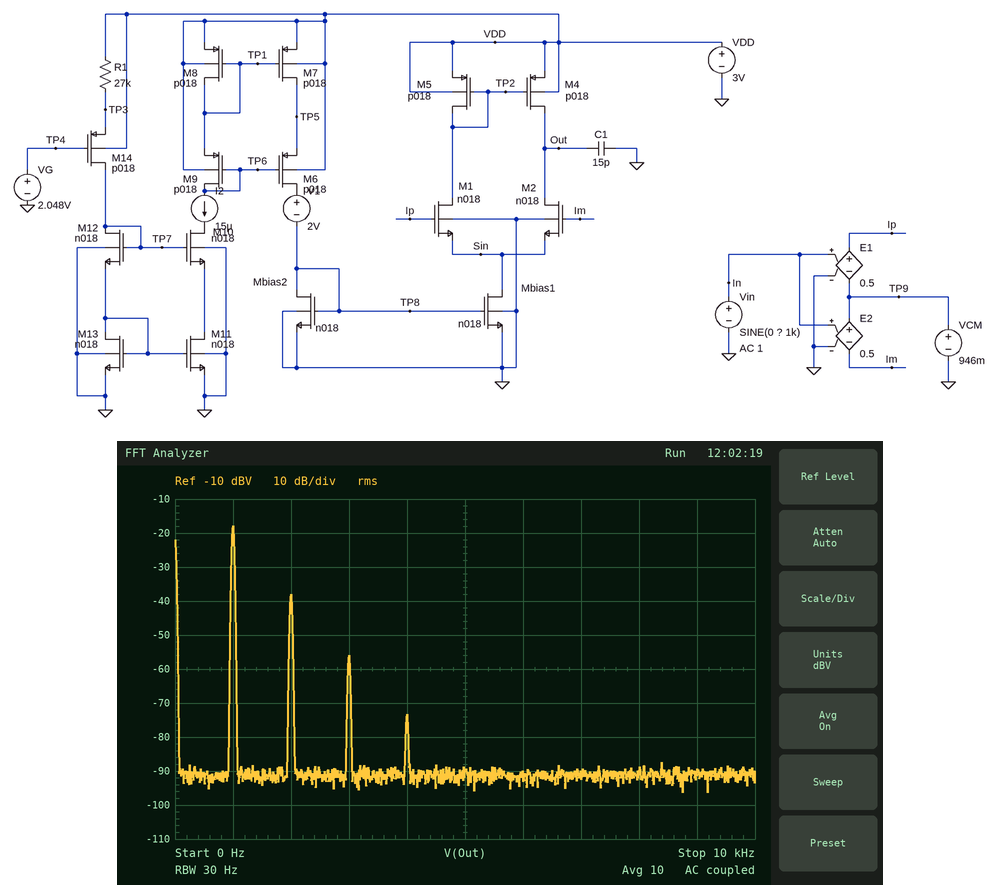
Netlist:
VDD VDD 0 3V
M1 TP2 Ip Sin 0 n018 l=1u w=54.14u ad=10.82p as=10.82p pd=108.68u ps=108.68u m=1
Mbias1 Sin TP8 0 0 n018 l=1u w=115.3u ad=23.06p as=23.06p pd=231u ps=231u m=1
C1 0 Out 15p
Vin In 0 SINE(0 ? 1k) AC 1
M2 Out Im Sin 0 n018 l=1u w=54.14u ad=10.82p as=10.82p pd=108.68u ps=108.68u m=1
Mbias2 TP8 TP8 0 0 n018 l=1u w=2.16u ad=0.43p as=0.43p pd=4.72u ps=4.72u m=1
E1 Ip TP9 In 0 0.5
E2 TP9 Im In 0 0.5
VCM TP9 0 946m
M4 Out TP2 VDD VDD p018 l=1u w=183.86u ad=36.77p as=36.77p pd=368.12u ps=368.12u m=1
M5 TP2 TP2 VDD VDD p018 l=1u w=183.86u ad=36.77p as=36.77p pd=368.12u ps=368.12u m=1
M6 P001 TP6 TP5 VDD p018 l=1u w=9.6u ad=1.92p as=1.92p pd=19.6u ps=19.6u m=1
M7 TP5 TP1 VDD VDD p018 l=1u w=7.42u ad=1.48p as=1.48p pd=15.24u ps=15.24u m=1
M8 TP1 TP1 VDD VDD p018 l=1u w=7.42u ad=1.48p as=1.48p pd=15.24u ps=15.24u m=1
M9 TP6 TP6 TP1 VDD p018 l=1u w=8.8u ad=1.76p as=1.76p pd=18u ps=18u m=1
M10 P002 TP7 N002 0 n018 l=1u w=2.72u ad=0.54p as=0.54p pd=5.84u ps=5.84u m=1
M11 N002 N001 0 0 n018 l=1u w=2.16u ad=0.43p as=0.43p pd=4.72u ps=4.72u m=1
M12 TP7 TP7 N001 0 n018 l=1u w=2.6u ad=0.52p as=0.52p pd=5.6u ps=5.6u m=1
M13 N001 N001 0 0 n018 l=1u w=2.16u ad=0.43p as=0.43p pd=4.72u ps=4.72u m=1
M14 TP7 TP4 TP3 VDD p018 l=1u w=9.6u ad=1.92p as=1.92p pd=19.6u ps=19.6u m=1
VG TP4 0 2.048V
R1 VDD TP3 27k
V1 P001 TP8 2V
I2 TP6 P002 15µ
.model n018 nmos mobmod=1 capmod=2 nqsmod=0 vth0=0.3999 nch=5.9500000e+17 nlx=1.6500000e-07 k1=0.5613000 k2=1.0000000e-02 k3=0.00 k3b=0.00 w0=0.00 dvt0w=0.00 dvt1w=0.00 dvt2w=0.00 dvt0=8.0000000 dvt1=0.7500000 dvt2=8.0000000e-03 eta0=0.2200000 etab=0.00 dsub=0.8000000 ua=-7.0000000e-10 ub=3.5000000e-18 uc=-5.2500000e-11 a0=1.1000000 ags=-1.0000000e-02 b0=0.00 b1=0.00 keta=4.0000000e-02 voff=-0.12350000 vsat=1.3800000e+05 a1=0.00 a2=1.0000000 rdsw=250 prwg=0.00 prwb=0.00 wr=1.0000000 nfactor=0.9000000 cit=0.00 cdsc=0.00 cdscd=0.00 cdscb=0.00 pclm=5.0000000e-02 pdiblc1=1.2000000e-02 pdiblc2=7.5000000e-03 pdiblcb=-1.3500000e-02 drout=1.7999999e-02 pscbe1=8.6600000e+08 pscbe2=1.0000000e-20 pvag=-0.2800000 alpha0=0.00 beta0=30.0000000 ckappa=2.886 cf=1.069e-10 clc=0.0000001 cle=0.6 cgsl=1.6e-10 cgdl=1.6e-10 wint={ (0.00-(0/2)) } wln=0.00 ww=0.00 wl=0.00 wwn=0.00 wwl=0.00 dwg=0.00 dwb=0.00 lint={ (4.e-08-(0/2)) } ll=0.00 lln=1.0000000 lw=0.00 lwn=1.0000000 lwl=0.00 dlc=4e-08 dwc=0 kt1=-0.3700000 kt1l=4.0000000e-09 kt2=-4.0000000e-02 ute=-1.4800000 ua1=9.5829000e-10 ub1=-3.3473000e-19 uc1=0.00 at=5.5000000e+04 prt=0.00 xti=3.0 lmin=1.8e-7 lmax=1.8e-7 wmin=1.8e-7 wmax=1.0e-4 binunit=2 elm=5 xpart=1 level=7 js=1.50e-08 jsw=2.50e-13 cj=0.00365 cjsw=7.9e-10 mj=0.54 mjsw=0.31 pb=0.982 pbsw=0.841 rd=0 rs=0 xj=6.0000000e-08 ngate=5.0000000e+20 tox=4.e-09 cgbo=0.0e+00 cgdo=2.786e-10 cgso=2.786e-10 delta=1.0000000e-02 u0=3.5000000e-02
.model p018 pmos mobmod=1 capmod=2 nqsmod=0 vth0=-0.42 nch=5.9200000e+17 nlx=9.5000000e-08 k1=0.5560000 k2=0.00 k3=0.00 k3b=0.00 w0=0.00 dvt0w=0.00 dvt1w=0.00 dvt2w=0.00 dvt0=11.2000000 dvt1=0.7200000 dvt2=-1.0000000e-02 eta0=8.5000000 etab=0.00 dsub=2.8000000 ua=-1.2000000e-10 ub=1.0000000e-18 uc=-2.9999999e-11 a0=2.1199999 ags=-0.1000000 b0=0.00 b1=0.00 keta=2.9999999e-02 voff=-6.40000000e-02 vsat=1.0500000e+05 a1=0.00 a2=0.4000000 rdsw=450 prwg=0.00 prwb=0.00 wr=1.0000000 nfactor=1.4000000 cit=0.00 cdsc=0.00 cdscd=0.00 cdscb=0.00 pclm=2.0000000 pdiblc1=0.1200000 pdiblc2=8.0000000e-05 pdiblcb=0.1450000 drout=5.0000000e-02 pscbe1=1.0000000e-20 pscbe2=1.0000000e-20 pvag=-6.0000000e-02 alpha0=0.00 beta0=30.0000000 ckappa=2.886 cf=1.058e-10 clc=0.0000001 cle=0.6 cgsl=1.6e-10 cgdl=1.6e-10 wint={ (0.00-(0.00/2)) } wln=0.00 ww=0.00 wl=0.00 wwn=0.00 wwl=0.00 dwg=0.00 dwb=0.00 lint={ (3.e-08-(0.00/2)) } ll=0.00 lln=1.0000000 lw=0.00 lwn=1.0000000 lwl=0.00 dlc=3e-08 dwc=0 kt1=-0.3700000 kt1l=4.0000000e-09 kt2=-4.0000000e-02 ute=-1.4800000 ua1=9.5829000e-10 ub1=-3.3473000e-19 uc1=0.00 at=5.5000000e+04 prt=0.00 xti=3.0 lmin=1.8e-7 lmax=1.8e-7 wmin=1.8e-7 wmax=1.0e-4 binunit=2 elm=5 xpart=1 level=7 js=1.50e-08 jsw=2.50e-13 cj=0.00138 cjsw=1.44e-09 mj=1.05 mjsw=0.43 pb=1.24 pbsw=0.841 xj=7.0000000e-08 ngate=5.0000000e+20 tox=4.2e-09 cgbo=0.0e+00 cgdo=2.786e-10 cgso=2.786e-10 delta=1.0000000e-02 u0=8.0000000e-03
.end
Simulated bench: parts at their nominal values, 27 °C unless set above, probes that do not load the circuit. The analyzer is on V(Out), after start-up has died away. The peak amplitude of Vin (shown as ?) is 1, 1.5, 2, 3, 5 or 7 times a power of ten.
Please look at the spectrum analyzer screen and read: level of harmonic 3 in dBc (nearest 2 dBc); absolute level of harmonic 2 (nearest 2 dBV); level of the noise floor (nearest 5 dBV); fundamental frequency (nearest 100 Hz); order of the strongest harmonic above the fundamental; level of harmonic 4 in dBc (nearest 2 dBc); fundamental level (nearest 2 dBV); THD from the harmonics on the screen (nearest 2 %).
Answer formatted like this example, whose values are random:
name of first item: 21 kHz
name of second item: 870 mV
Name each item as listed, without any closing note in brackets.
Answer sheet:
level of harmonic 3 in dBc: -38 dBc
absolute level of harmonic 2: -38 dBV
level of the noise floor: -90 dBV
fundamental frequency: 1.0 kHz
order of the strongest harmonic above the fundamental: 2
level of harmonic 4 in dBc: -56 dBc
fundamental level: -18 dBV
THD from the harmonics on the screen: 10 %
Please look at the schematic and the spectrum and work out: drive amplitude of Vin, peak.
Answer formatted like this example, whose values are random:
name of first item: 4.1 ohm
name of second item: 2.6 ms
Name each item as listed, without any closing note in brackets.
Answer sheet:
drive amplitude of Vin, peak: 5 mV
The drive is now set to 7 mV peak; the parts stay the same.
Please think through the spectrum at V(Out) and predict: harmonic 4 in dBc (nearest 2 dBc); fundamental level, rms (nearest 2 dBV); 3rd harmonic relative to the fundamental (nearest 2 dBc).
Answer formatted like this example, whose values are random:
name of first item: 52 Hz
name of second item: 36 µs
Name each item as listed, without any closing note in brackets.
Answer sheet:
harmonic 4 in dBc: -48 dBc
fundamental level, rms: -14 dBV
3rd harmonic relative to the fundamental: -32 dBc
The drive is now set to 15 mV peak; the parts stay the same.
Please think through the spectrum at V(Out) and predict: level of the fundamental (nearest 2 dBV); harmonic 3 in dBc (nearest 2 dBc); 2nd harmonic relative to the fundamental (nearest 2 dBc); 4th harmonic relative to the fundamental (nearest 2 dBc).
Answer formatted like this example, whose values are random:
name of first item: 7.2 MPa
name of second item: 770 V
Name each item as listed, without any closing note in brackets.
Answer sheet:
level of the fundamental: -6 dBV
harmonic 3 in dBc: -26 dBc
2nd harmonic relative to the fundamental: -12 dBc
4th harmonic relative to the fundamental: -38 dBc
